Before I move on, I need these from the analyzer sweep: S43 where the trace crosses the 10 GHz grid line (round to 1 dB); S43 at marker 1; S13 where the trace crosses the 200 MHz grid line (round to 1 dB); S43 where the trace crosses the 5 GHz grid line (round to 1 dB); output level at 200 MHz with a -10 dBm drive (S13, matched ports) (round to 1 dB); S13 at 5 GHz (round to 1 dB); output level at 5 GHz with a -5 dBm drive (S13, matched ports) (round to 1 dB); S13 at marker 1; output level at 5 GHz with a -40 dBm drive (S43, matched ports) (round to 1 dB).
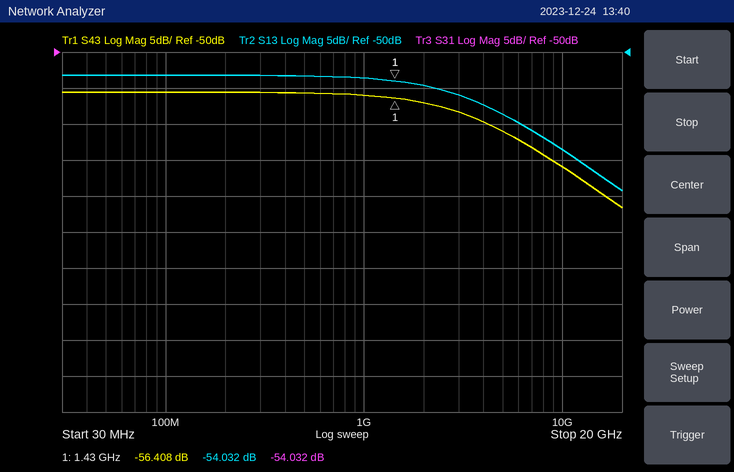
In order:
-66 dB
-56.408 dB
-53 dB
-61 dB
-63 dBm
-59 dB
-64 dBm
-54.032 dB
-101 dBm
